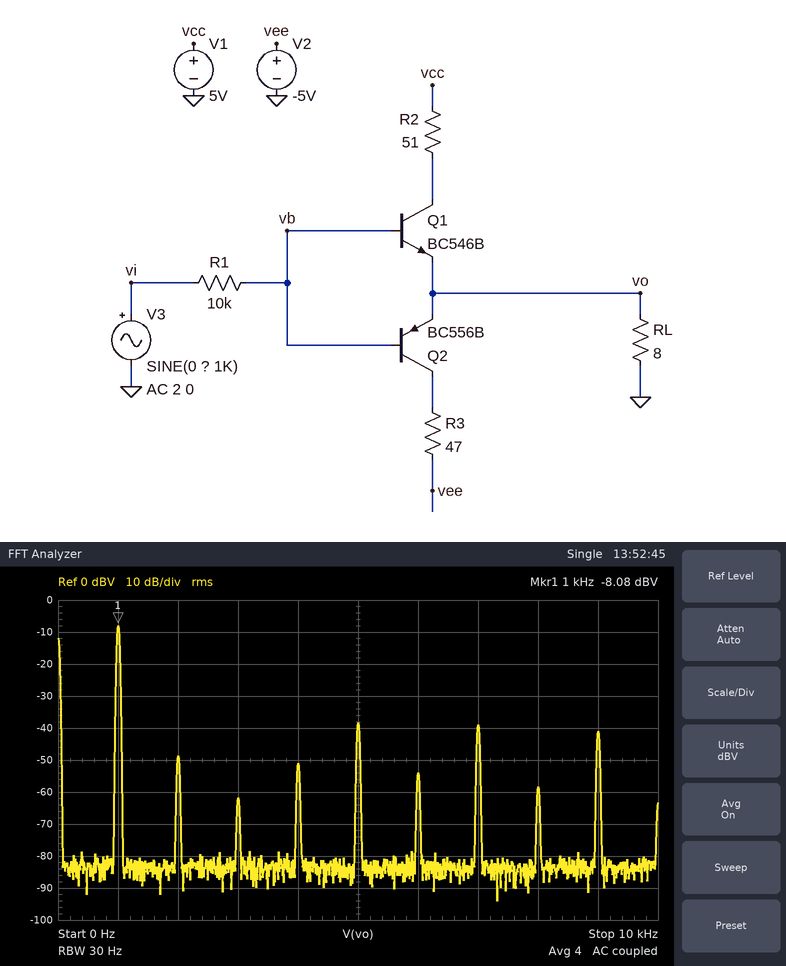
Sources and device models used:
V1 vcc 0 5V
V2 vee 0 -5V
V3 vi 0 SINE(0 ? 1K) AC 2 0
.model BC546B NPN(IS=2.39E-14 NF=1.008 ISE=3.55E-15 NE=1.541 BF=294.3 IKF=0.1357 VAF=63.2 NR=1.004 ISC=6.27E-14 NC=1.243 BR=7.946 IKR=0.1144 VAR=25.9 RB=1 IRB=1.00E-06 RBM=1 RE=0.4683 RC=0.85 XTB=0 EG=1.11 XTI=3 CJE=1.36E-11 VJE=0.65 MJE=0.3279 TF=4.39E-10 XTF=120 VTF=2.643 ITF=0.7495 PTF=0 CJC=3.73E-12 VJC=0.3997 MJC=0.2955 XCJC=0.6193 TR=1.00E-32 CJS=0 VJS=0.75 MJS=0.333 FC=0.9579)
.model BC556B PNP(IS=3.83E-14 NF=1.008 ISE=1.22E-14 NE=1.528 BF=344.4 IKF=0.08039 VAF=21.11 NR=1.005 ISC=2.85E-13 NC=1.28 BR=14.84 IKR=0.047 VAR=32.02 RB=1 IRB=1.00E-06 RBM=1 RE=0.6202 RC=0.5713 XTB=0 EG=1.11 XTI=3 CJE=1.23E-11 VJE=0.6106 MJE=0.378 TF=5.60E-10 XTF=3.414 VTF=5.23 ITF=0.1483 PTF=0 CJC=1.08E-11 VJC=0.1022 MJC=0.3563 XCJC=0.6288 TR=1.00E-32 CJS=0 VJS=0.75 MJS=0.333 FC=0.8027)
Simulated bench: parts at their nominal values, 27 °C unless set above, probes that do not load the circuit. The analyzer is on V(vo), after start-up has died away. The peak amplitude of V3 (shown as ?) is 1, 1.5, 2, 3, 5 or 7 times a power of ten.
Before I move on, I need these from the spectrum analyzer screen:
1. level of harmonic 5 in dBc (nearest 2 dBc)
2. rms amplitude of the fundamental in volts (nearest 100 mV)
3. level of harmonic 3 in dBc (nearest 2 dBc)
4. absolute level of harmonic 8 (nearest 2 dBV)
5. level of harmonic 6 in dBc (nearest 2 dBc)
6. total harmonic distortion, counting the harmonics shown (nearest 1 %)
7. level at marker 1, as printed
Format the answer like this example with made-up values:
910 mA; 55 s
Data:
-30 dBc; 400 mV; -54 dBc; -58 dBV; -46 dBc; 5 %; -8.08 dBV
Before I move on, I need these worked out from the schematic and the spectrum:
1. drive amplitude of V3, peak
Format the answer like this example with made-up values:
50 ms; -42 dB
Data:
5 V
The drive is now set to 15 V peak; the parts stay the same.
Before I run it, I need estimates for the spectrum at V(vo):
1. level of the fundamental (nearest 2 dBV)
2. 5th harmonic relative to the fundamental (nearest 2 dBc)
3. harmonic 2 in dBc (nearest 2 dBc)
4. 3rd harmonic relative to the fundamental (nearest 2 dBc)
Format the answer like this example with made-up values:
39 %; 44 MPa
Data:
-4 dBV; -22 dBc; -38 dBc; -12 dBc
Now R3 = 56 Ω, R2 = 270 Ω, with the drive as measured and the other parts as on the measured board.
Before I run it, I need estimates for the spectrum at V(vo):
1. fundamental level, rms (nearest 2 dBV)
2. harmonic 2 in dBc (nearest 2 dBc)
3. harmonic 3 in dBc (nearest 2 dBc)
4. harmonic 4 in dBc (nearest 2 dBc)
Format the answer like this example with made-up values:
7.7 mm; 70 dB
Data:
-12 dBV; -12 dBc; -22 dBc; -26 dBc
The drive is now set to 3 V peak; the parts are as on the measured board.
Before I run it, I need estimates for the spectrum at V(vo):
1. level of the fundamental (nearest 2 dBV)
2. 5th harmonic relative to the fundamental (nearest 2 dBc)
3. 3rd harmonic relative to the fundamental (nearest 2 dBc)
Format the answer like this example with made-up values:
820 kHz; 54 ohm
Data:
-12 dBV; -24 dBc; -22 dBc
